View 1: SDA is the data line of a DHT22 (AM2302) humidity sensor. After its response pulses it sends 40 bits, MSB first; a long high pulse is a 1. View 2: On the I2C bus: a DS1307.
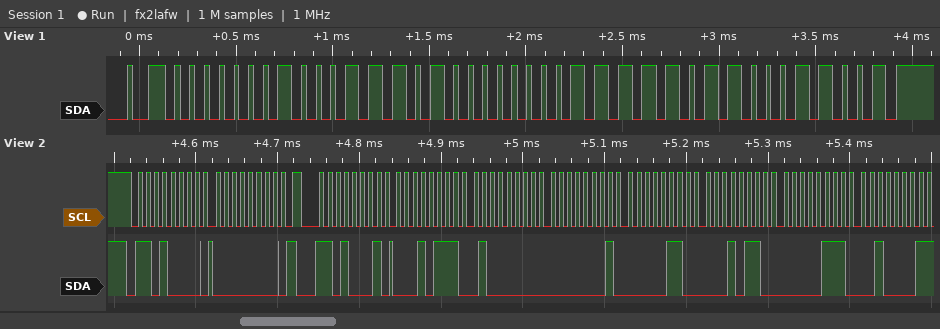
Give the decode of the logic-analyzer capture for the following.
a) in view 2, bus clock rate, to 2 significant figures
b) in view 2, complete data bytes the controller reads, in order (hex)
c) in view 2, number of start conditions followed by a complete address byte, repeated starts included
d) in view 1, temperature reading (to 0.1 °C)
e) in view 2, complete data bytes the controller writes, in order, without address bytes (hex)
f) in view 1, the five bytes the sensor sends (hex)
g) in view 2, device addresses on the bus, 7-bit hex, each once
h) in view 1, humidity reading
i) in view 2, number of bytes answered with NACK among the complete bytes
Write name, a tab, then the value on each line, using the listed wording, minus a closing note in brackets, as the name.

in view 2, bus clock rate, to 2 significant figures	100 kHz
in view 2, complete data bytes the controller reads, in order	17 40 01 06 16 07 21
in view 2, number of start conditions followed by a complete address byte, repeated starts included	2
in view 1, temperature reading	25.1 °C
in view 2, complete data bytes the controller writes, in order, without address bytes	00
in view 1, the five bytes the sensor sends	01 1D 00 FB 19
in view 2, device addresses on the bus, 7-bit hex, each once	0x68
in view 1, humidity reading	28.5 %
in view 2, number of bytes answered with NACK among the complete bytes	1
